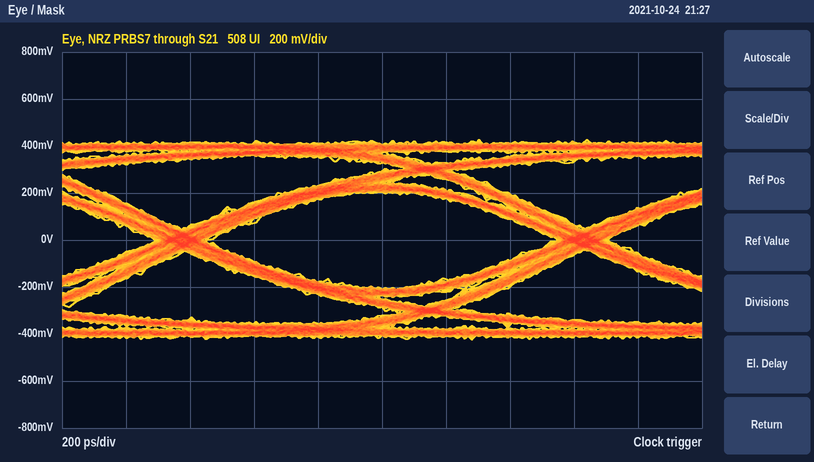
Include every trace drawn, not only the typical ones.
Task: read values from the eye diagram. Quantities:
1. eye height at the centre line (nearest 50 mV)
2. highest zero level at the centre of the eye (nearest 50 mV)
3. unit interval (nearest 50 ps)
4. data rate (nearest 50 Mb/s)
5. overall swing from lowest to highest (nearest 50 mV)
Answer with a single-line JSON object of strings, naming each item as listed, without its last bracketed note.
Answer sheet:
{"eye height at the centre line": "400 mV", "highest zero level at the centre of the eye": "-200 mV", "unit interval": "1.25 ns", "data rate": "800 Mb/s", "overall swing from lowest to highest": "850 mV"}
